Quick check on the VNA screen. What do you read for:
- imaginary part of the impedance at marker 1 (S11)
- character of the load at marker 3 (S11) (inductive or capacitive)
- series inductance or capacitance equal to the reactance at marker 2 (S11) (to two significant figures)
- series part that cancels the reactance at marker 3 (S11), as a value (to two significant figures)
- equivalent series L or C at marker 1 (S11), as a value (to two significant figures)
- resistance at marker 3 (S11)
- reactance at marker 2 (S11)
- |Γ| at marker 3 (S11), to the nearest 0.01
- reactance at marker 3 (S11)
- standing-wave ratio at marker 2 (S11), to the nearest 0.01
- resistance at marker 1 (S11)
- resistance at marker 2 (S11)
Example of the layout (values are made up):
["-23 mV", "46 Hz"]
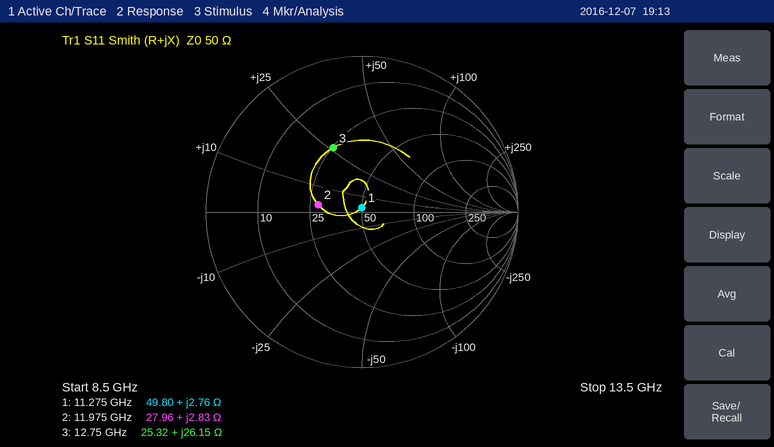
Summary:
["+2.76 Ω", "inductive", "38 pH", "480 fF", "39 pH", "25.32 Ω", "+2.83 Ω", "0.45", "+26.15 Ω", "1.80", "49.80 Ω", "27.96 Ω"]
